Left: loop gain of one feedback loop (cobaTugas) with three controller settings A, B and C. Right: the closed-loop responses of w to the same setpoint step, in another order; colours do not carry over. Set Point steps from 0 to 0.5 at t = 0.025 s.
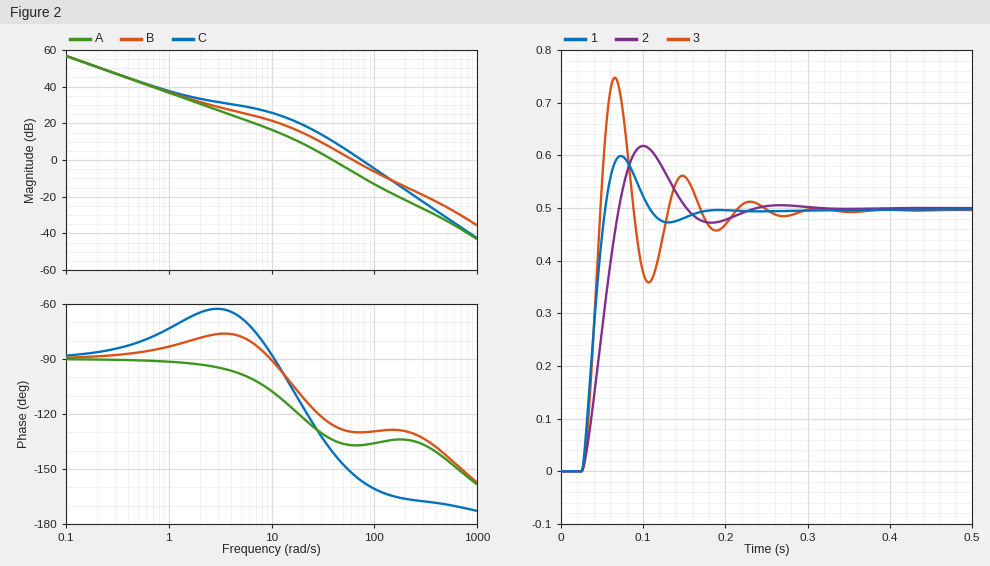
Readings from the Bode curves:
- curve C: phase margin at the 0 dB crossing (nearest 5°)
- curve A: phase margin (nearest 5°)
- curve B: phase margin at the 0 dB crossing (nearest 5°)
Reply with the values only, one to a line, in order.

25°
45°
50°
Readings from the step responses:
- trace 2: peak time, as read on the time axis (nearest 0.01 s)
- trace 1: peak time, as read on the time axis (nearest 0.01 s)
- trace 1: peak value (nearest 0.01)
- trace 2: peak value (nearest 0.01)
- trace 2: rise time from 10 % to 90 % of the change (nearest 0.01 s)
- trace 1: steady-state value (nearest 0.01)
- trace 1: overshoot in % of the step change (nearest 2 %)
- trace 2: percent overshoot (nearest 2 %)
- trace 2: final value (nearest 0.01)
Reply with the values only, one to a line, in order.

0.10 s
0.07 s
0.60
0.62
0.03 s
0.50
20 %
24 %
0.50
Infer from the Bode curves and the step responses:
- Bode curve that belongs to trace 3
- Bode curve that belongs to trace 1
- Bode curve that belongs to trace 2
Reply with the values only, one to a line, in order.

C
B
A
